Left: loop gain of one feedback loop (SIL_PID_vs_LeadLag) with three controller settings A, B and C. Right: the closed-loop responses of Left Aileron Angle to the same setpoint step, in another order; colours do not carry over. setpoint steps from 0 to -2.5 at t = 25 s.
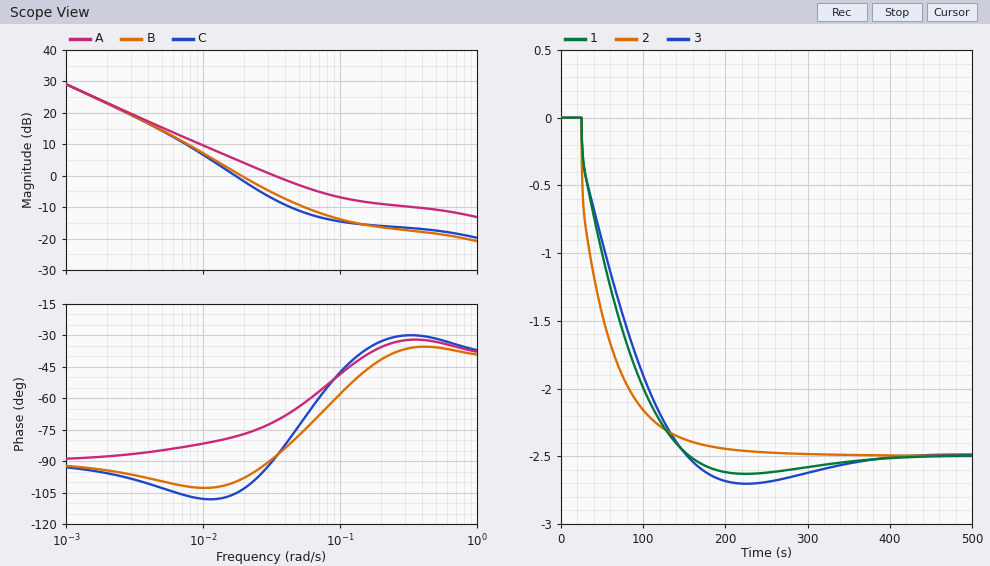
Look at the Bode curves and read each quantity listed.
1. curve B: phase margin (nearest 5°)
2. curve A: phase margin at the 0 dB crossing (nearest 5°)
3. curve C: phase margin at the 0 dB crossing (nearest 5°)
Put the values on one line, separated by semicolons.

80°; 110°; 75°
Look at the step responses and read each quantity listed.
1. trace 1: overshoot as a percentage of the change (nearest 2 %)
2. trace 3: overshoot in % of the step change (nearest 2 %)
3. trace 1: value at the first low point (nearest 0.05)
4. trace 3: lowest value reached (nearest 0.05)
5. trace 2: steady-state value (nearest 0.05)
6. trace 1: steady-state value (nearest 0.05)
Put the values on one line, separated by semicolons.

6 %; 8 %; -2.65; -2.70; -2.50; -2.50
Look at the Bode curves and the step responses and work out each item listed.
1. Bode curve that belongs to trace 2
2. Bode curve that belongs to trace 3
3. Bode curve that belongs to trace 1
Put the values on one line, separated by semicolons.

A; C; B
